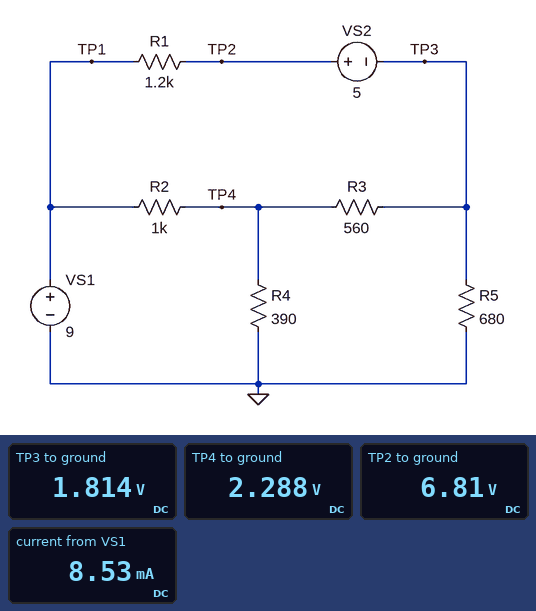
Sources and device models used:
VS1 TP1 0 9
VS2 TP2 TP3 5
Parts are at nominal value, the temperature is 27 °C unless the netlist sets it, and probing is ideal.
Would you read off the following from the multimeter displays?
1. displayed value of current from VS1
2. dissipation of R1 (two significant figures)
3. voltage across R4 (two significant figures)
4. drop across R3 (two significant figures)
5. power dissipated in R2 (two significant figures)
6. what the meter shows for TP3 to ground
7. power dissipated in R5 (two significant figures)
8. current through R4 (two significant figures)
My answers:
8.53 mA
4.0 mW
2.3 V
470 mV
45 mW
1.814 V
4.8 mW
5.9 mA
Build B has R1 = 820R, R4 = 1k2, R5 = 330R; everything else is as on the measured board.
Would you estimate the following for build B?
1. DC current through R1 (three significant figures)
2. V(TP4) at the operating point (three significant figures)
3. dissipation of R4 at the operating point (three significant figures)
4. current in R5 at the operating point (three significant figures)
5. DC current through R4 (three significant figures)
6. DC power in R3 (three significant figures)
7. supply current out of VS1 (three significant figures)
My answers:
2.67 mA
3.38 V
9.51 mW
5.48 mA
2.82 mA
4.41 mW
8.29 mA
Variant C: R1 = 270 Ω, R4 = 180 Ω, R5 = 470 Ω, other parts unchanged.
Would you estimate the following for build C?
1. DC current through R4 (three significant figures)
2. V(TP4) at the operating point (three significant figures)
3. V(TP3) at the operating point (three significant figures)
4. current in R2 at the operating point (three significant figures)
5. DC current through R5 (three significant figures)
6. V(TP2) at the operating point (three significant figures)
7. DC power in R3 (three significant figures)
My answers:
8.75 mA
1.57 V
2.31 V
7.43 mA
4.92 mA
7.31 V
977 µW
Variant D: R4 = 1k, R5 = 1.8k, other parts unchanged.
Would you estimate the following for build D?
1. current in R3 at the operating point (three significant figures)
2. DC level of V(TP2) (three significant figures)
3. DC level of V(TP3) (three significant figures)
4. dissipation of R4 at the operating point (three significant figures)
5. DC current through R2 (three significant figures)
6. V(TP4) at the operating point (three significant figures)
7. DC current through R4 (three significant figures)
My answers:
1.18 mA
8.25 V
3.25 V
15.3 mW
5.09 mA
3.91 V
3.91 mA
